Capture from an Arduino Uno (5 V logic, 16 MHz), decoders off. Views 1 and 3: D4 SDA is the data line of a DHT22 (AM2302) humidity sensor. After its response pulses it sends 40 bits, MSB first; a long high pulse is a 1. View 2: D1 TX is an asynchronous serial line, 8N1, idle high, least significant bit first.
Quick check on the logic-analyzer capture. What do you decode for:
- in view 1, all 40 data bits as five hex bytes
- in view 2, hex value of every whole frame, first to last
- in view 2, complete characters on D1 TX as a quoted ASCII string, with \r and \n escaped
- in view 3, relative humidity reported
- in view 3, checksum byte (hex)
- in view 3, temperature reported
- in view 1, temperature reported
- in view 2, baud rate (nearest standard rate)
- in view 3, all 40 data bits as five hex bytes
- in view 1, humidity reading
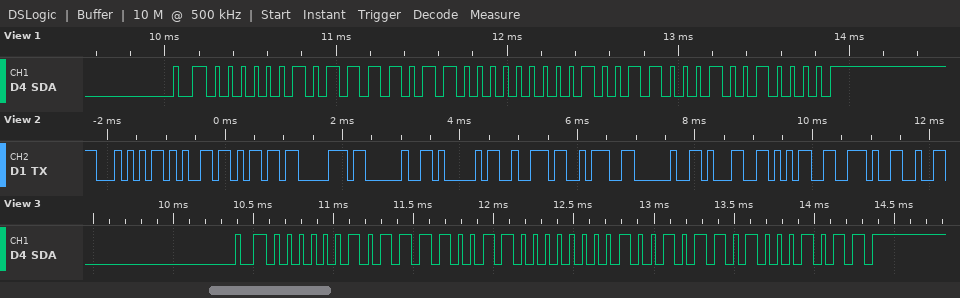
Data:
02 F6 00 98 90
0x54 0x65 0x6D 0x70 0x20 0x41 0x72 0x3A 0x20 0x31 0x35 0x2E
"Temp Ar: 15."
75.5 %
0x8B
15.0 °C
15.2 °C
9600 baud
02 F3 00 96 8B
75.8 %
